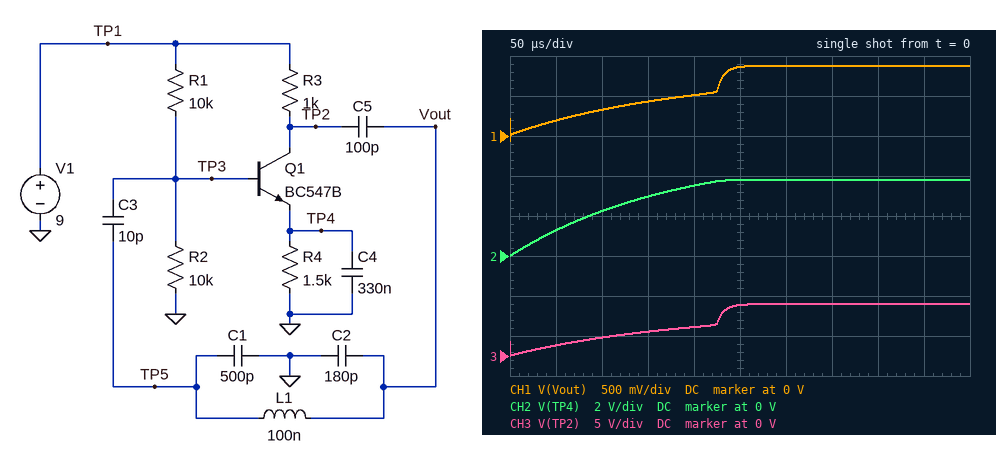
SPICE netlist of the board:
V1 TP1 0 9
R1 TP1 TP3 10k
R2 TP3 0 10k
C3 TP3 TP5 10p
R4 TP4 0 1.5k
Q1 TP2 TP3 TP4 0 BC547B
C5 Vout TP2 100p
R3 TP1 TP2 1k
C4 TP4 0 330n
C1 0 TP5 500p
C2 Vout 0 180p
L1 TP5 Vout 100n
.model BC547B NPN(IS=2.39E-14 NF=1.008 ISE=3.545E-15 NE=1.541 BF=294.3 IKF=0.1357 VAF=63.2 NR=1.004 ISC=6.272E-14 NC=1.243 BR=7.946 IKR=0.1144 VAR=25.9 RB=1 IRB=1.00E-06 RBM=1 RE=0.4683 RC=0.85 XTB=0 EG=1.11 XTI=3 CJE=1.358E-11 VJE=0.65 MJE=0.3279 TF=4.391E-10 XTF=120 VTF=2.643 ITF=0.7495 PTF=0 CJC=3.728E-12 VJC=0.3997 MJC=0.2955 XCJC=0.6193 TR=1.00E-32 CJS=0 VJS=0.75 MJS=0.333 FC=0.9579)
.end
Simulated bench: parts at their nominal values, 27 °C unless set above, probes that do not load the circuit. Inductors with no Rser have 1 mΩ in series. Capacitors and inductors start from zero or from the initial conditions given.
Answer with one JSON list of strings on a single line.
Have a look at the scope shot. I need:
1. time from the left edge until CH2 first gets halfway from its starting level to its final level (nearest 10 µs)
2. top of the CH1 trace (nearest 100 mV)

["80 µs", "900 mV"]
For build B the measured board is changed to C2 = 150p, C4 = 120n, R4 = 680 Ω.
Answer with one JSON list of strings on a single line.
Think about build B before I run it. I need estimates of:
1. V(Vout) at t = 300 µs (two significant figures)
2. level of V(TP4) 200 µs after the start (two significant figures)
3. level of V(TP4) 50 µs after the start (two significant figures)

["550 mV", "3.6 V", "2.4 V"]
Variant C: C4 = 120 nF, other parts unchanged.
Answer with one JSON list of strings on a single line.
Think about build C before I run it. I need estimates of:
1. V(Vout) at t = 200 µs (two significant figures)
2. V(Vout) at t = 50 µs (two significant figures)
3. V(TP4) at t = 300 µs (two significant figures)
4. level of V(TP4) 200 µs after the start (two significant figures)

["880 mV", "410 mV", "3.8 V", "3.8 V"]
